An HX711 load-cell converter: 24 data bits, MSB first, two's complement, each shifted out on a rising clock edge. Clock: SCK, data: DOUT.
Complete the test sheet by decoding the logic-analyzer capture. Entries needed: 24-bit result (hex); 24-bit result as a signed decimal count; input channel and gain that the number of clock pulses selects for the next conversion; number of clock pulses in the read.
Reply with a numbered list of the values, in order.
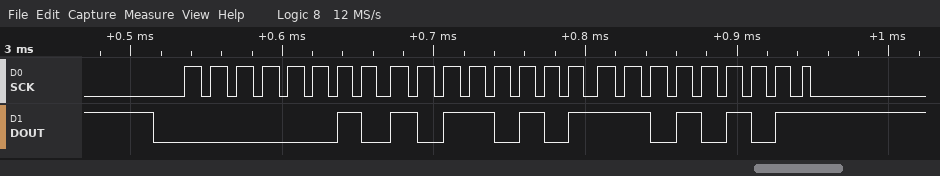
1. 0x02B5D5
2. 177621
3. channel A, gain 128
4. 25
